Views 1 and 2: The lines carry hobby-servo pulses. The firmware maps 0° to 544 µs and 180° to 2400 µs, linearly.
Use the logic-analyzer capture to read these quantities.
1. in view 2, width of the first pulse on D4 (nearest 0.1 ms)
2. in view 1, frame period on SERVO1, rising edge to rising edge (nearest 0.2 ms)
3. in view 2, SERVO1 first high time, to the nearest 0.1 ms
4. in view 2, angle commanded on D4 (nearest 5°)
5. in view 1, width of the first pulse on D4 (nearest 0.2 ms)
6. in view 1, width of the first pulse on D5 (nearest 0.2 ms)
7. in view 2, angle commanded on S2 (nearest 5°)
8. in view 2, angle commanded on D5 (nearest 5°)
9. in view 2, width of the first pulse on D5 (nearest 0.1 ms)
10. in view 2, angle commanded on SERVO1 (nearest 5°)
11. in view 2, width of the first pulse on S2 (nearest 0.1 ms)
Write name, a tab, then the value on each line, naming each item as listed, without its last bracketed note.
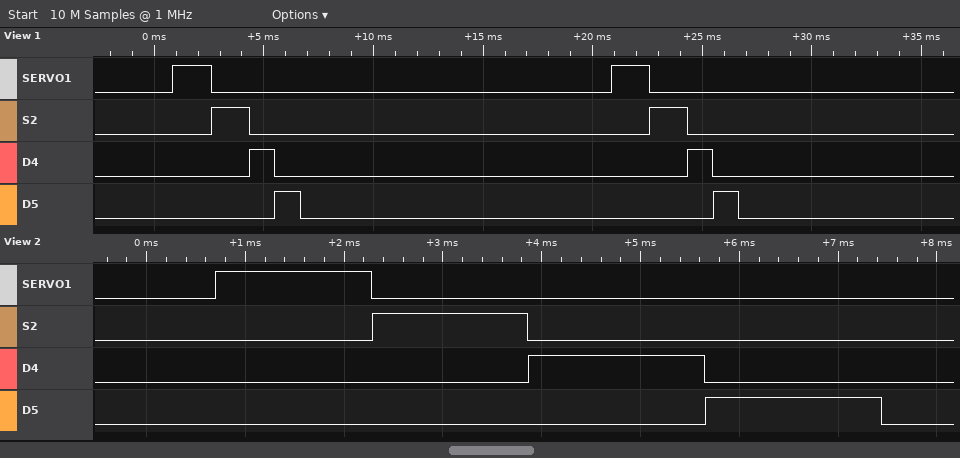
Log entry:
in view 2, width of the first pulse on D4	1.8 ms
in view 1, frame period on SERVO1, rising edge to rising edge	20.0 ms
in view 2, SERVO1 first high time, to the nearest 0.1 ms	1.6 ms
in view 2, angle commanded on D4	120°
in view 1, width of the first pulse on D4	1.2 ms
in view 1, width of the first pulse on D5	1.2 ms
in view 2, angle commanded on S2	100°
in view 2, angle commanded on D5	120°
in view 2, width of the first pulse on D5	1.8 ms
in view 2, angle commanded on SERVO1	100°
in view 2, width of the first pulse on S2	1.6 ms
